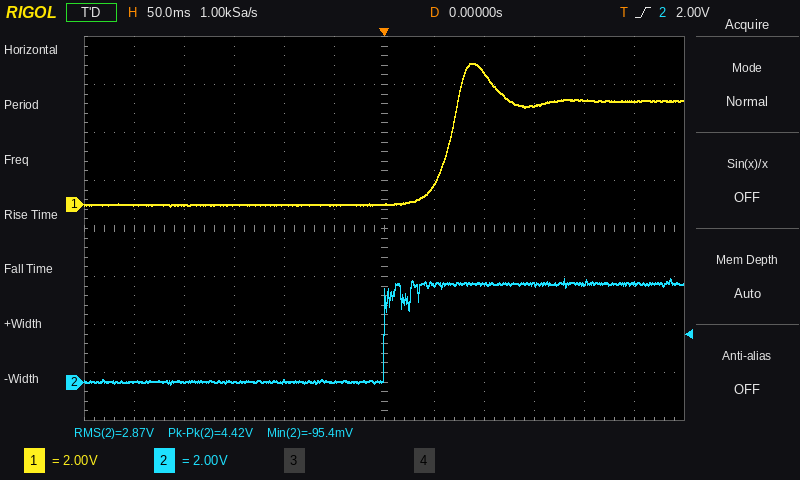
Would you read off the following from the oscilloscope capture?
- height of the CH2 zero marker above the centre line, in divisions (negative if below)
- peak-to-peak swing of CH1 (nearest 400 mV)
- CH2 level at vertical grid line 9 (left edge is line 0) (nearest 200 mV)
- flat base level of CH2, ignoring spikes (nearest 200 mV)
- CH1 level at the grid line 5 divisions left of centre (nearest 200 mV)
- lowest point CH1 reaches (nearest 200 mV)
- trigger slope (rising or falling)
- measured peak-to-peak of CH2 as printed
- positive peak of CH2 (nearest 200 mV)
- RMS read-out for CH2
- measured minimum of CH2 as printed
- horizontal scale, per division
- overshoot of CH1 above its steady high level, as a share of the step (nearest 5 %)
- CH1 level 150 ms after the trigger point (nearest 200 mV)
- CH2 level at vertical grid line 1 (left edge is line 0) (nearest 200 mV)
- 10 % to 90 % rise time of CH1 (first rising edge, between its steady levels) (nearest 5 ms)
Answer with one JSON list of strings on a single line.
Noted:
["-3.2 div", "6.0 V", "4.0 V", "0.0 V", "0.0 V", "0.0 V", "rising", "4.42 V", "4.4 V", "2.87 V", "-95.4 mV", "50 ms", "35 %", "4.2 V", "0.0 V", "30 ms"]
